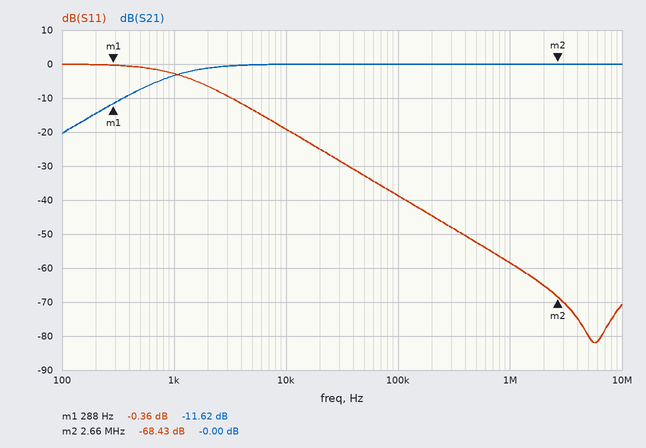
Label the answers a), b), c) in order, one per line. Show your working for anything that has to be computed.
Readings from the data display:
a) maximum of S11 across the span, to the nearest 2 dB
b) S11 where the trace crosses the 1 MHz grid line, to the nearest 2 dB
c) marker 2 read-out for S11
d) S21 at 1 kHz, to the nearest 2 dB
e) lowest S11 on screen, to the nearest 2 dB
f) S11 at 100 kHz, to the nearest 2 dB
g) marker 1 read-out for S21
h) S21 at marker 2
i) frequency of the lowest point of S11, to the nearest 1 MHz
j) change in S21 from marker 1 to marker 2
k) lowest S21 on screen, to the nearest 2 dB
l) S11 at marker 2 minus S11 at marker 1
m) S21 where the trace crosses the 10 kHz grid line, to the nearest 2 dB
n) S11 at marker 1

a) 0 dB
b) -58 dB
c) -68.43 dB
d) -4 dB
e) -82 dB
f) -38 dB
g) -11.62 dB
h) -0.00 dB
i) 6 MHz
j) -0 − (-11.62) = 11.62 dB
k) -20 dB
l) -68.43 − (-0.36) = -68.07 dB
m) 0 dB
n) -0.36 dB
